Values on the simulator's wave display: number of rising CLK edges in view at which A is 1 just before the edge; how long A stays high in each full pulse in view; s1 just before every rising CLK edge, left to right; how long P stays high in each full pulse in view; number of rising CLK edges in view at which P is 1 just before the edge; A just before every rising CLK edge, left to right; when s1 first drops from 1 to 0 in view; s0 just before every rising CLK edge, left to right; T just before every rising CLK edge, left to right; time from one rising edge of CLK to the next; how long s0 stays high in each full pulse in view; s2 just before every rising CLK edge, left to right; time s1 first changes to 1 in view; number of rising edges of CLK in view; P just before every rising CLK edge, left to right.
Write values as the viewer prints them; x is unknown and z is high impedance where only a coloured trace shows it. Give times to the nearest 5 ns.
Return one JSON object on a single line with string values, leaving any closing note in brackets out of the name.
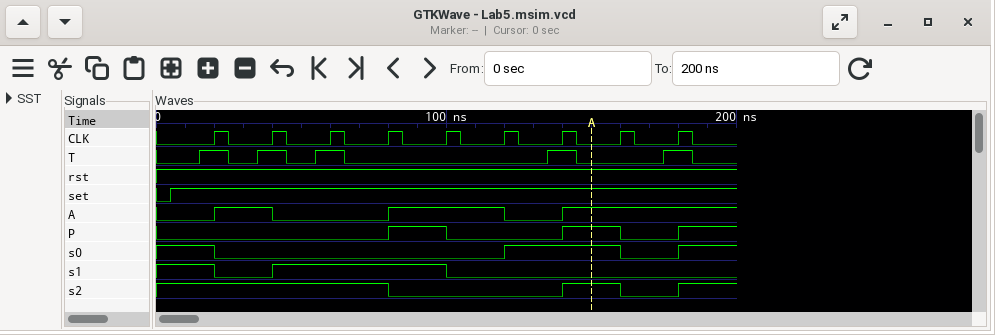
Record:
{"number of rising CLK edges in view at which A is 1 just before the edge": "5", "how long A stays high in each full pulse in view": "20 ns, 40 ns", "s1 just before every rising CLK edge, left to right": "1 0 1 1 1 0 0 0 0", "how long P stays high in each full pulse in view": "20 ns, 20 ns", "number of rising CLK edges in view at which P is 1 just before the edge": "2", "A just before every rising CLK edge, left to right": "0 1 0 0 1 1 0 1 1", "when s1 first drops from 1 to 0 in view": "20 ns", "s0 just before every rising CLK edge, left to right": "1 0 0 0 0 0 1 1 0", "T just before every rising CLK edge, left to right": "1 1 1 0 0 0 1 0 1", "time from one rising edge of CLK to the next": "20 ns", "how long s0 stays high in each full pulse in view": "40 ns", "s2 just before every rising CLK edge, left to right": "1 1 1 1 0 0 0 1 0", "time s1 first changes to 1 in view": "40 ns", "number of rising edges of CLK in view": "9", "P just before every rising CLK edge, left to right": "0 0 0 0 1 0 0 1 0"}
